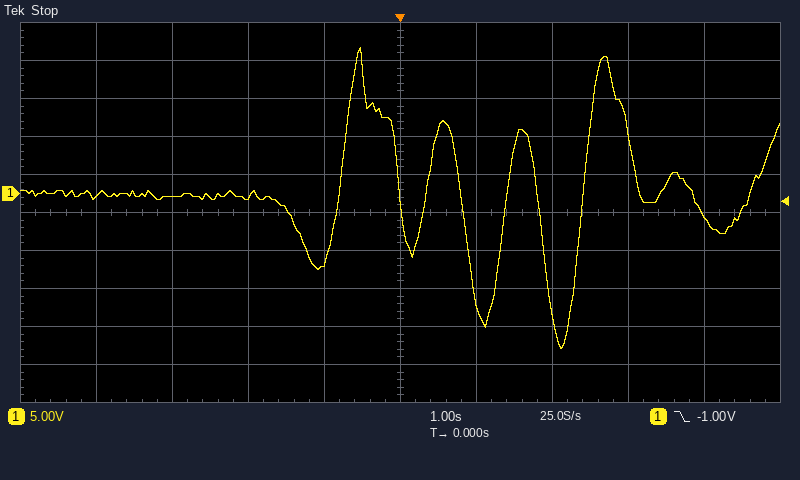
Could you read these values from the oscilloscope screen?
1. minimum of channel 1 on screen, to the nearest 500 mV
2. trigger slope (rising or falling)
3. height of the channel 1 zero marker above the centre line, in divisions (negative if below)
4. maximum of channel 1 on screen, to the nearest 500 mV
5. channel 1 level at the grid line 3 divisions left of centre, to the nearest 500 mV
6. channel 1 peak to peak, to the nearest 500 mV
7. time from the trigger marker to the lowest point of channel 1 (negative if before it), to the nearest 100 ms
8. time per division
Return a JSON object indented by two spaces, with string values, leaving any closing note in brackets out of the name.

{
  "minimum of channel 1 on screen, to the nearest 500 mV": "-20.5 V",
  "trigger slope": "falling",
  "height of the channel 1 zero marker above the centre line, in divisions": "+0.5 div",
  "maximum of channel 1 on screen, to the nearest 500 mV": "19.0 V",
  "channel 1 level at the grid line 3 divisions left of centre, to the nearest 500 mV": "-500 mV",
  "channel 1 peak to peak, to the nearest 500 mV": "39.5 V",
  "time from the trigger marker to the lowest point of channel 1 (negative if before it), to the nearest 100 ms": "+2.1 s",
  "time per division": "1 s"
}
